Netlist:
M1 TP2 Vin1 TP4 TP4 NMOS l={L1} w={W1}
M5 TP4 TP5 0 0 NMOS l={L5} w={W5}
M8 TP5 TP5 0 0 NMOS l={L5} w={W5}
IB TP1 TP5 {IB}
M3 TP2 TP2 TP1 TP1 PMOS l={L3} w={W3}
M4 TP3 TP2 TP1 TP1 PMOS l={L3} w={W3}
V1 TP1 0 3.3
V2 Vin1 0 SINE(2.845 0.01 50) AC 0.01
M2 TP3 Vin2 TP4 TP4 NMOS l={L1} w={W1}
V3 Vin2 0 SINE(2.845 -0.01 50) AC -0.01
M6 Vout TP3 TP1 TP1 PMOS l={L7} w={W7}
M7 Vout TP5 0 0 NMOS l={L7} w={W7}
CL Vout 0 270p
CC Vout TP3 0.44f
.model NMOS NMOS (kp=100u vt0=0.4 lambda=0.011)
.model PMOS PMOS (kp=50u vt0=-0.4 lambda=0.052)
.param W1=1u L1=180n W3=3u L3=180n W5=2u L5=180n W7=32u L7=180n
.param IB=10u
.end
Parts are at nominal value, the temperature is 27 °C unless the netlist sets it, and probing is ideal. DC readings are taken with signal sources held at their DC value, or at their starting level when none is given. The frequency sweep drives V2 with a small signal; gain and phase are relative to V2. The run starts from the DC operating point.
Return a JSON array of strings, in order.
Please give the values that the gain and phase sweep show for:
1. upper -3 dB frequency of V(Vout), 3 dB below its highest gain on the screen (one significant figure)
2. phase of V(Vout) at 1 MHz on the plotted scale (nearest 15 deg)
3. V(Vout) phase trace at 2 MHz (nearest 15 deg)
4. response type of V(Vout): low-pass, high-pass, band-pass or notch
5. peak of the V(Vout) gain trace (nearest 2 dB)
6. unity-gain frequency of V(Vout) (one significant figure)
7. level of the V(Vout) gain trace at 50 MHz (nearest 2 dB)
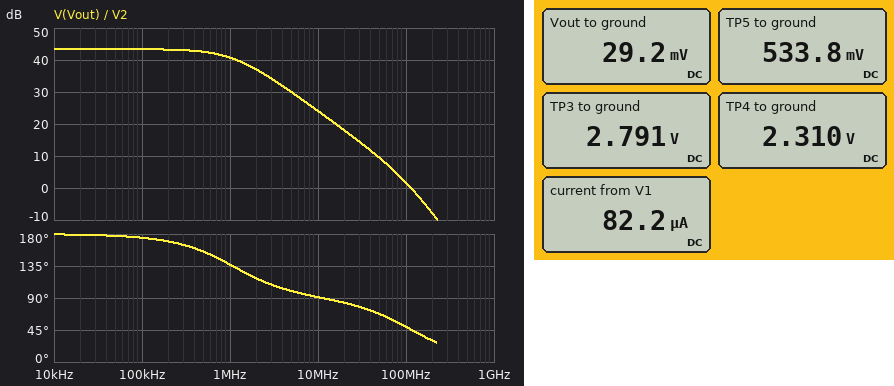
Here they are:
["1 MHz", "135 deg", "120 deg", "low-pass", "44 dB", "100 MHz", "10 dB"]
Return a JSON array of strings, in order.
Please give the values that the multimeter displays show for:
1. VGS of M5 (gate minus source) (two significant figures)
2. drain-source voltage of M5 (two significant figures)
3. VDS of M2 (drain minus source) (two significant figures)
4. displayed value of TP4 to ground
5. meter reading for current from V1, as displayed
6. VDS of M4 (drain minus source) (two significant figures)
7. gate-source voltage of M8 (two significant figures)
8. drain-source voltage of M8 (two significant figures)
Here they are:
["530 mV", "2.3 V", "480 mV", "2.310 V", "82.2 µA", "-510 mV", "530 mV", "530 mV"]
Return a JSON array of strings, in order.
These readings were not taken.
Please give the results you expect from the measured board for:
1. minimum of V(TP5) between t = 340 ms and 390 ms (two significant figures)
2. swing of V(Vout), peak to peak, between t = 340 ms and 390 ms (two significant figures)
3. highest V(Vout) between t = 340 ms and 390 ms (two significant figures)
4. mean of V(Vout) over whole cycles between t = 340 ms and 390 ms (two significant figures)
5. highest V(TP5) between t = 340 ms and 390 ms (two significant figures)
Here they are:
["530 mV", "3.3 V", "3.3 V", "1.6 V", "530 mV"]
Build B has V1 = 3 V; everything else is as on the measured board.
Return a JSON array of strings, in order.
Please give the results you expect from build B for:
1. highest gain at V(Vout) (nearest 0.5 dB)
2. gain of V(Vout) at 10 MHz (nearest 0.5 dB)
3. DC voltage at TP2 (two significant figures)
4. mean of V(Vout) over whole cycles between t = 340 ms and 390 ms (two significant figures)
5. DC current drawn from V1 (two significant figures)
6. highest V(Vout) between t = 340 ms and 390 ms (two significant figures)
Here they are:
["43.0 dB", "24.0 dB", "2.5 V", "1.3 V", "81 µA", "2.9 V"]
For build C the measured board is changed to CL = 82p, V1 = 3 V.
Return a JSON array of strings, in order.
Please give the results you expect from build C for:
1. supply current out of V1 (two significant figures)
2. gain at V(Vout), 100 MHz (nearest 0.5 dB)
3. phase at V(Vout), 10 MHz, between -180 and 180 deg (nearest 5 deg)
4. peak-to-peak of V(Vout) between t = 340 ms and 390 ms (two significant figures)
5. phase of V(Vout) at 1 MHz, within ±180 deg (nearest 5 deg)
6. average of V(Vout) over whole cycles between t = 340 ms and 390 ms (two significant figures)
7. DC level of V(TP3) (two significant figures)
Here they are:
["81 µA", "12.0 dB", "105 deg", "2.9 V", "165 deg", "1.3 V", "2.5 V"]
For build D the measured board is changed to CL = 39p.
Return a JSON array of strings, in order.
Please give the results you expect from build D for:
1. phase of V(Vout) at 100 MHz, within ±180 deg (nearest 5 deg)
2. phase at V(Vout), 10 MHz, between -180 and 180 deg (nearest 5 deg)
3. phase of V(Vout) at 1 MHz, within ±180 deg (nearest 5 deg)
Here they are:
["55 deg", "120 deg", "170 deg"]
